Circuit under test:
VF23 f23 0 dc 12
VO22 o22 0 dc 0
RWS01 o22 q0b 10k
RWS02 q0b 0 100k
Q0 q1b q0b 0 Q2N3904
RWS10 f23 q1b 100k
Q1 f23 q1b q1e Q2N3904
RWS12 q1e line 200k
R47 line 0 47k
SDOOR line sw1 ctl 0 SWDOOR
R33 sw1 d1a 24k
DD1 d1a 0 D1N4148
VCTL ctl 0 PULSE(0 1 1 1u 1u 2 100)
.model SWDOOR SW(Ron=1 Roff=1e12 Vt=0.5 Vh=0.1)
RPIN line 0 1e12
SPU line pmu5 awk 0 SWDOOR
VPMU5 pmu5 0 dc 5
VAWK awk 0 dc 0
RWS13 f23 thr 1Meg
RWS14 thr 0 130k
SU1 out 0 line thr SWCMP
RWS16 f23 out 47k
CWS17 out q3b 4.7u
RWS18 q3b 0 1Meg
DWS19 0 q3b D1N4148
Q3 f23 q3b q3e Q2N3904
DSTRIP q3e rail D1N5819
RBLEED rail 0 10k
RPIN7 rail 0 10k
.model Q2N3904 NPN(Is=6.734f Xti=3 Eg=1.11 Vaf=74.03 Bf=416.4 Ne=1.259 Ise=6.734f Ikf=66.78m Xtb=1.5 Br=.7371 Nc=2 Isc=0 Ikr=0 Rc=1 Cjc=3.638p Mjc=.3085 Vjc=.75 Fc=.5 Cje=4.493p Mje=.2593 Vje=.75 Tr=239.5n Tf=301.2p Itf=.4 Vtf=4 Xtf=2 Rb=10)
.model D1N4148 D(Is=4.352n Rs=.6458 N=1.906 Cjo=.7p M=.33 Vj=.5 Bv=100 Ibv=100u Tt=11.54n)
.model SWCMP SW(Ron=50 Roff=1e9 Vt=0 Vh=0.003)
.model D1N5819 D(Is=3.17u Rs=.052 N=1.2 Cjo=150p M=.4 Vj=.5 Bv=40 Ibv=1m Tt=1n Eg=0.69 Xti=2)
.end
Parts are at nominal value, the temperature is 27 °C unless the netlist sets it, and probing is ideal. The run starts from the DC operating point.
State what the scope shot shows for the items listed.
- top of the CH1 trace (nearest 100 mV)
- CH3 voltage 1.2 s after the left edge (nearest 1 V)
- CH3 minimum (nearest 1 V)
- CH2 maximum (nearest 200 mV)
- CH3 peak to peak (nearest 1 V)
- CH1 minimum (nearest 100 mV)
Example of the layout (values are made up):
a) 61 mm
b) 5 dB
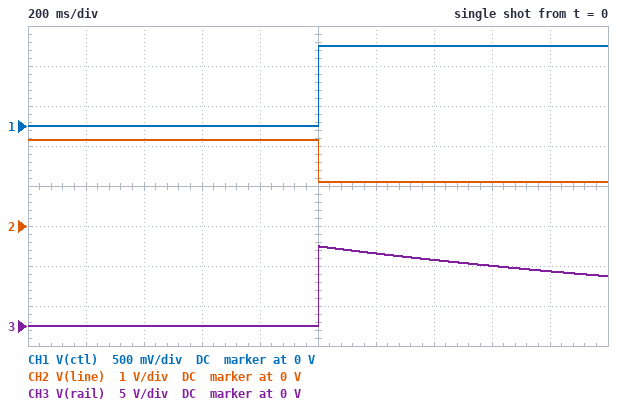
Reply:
a) 1.0 V
b) 9 V
c) 0 V
d) 2.2 V
e) 10 V
f) 0 V
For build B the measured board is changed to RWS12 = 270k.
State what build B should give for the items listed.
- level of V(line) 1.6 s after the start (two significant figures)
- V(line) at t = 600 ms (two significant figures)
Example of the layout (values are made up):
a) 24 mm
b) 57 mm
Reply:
a) 890 mV
b) 1.7 V
